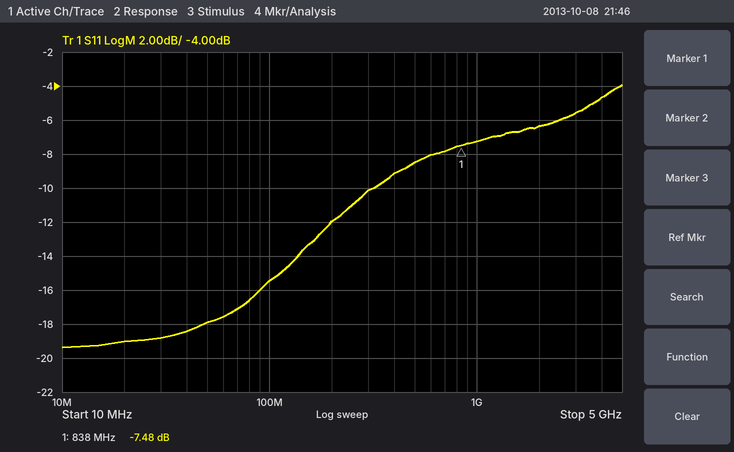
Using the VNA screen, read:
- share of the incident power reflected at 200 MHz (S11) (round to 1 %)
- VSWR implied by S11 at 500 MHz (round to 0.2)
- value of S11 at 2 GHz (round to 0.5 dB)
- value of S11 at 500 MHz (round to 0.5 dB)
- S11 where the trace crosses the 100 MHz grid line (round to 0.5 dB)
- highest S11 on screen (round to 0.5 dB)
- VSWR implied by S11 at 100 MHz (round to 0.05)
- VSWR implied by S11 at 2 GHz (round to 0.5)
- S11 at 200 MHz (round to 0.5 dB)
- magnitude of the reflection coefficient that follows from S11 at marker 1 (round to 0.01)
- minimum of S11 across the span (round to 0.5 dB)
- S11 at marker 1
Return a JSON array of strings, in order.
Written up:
["6 %", "2.2", "-6.5 dB", "-8.5 dB", "-15.5 dB", "-4.0 dB", "1.40", "3.0", "-12.0 dB", "0.42", "-19.5 dB", "-7.48 dB"]
